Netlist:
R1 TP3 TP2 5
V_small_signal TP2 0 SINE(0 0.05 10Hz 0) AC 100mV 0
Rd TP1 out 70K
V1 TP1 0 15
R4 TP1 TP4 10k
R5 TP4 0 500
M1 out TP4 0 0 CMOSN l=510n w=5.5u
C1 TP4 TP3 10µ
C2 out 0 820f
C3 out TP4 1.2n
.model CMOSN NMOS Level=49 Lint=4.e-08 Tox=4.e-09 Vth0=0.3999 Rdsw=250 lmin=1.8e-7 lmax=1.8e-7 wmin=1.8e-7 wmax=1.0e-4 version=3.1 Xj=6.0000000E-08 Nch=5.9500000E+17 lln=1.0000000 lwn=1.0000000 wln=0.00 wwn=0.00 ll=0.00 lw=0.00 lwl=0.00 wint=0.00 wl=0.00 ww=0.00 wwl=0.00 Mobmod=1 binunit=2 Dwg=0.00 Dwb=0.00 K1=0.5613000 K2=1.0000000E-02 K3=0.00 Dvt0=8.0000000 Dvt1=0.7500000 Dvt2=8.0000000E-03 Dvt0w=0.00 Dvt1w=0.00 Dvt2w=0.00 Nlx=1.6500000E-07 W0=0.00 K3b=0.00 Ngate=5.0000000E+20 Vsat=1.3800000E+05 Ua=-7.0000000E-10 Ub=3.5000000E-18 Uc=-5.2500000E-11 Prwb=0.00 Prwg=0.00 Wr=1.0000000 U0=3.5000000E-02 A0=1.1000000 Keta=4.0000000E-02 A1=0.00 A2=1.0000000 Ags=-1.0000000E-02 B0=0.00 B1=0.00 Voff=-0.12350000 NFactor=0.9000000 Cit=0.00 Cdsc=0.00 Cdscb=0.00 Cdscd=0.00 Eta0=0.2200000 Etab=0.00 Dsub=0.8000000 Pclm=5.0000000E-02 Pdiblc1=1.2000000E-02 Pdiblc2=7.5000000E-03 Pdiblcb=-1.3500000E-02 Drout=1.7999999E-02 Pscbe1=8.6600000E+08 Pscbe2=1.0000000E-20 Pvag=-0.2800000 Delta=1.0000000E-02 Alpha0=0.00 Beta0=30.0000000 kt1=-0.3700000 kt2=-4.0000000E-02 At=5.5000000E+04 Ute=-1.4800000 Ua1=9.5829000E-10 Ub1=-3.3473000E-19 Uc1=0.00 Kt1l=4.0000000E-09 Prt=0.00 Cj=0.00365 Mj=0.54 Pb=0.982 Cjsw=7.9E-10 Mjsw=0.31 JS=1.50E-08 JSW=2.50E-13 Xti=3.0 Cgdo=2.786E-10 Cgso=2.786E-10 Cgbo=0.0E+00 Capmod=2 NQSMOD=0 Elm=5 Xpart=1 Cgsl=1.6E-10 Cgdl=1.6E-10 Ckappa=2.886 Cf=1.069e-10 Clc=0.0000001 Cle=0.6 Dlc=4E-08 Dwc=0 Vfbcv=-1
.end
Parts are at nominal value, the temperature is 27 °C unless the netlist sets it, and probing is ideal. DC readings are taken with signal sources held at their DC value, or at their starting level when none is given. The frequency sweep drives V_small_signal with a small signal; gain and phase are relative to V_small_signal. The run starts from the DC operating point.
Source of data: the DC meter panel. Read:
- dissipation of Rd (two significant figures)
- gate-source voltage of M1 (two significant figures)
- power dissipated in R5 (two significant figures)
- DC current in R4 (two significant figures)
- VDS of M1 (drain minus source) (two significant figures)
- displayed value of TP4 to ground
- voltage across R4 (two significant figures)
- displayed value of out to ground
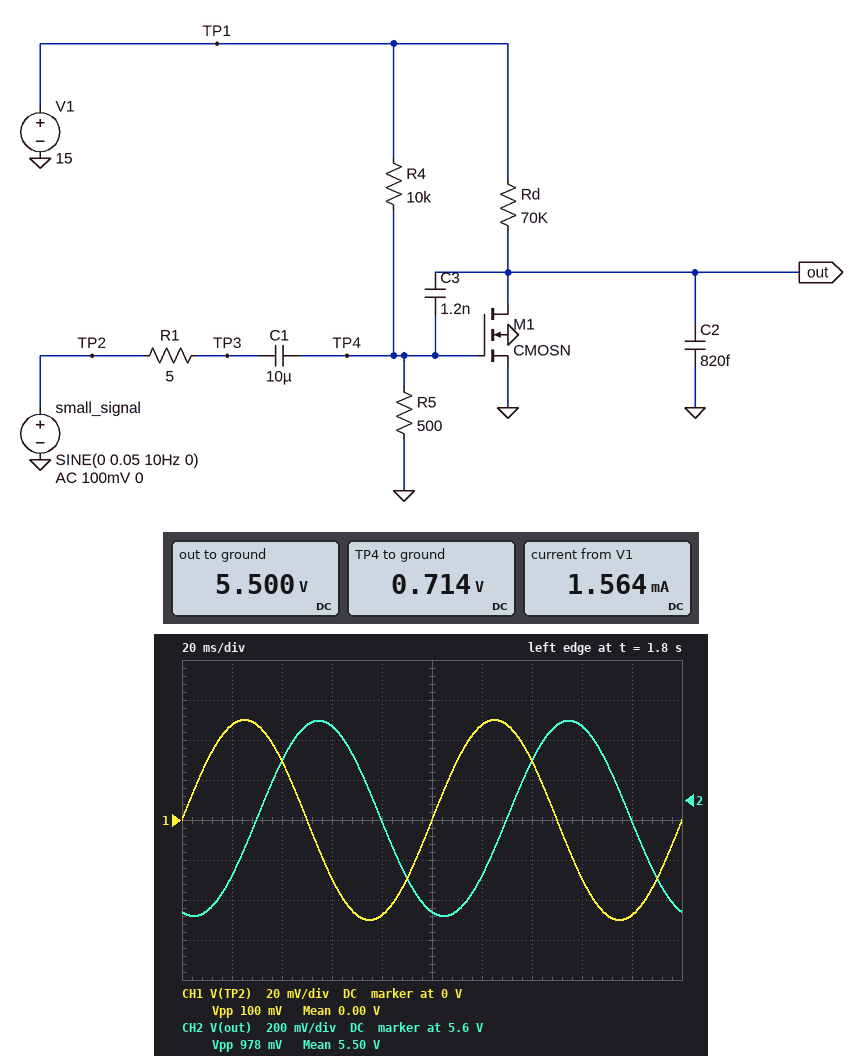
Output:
1.3 mW
710 mV
1.0 mW
1.4 mA
5.5 V
0.714 V
14 V
5.500 V
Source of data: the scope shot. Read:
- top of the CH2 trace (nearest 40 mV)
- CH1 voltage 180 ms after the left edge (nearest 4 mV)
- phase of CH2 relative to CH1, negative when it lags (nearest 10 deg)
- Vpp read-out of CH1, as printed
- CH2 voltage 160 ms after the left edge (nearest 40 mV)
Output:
6.00 V
-48 mV
-110 deg
100 mV
5.96 V
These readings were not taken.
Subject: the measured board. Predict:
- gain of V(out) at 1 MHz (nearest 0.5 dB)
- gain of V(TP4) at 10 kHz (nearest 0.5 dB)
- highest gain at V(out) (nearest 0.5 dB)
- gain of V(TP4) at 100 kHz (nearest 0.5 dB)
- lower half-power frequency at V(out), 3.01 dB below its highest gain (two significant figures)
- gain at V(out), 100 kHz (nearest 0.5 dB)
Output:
0 dB
0 dB
30.5 dB
0 dB
32 Hz
3.5 dB
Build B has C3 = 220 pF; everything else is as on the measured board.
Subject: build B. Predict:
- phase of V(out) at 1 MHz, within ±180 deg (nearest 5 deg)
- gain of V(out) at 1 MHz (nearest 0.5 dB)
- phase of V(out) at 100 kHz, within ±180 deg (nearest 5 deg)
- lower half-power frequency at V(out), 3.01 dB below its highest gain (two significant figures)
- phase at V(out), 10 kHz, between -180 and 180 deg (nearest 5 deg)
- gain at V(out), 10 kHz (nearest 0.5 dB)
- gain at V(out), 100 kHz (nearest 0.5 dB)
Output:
35 deg
1.5 dB
90 deg
33 Hz
150 deg
29.5 dB
16.0 dB
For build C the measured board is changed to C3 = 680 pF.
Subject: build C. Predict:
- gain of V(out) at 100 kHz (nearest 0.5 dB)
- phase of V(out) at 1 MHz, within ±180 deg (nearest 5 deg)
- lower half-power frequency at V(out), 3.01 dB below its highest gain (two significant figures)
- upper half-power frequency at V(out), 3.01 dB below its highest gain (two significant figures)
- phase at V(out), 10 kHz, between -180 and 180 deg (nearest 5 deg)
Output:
7.0 dB
10 deg
33 Hz
6.0 kHz
120 deg
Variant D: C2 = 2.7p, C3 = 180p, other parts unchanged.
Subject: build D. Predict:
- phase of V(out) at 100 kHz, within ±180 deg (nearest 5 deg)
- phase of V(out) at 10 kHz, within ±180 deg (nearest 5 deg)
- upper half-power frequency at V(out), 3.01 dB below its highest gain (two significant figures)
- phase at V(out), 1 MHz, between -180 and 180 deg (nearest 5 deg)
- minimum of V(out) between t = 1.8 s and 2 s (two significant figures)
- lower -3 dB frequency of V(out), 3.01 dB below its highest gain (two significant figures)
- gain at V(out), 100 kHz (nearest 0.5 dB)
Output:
95 deg
155 deg
22 kHz
40 deg
5.0 V
33 Hz
17.5 dB
